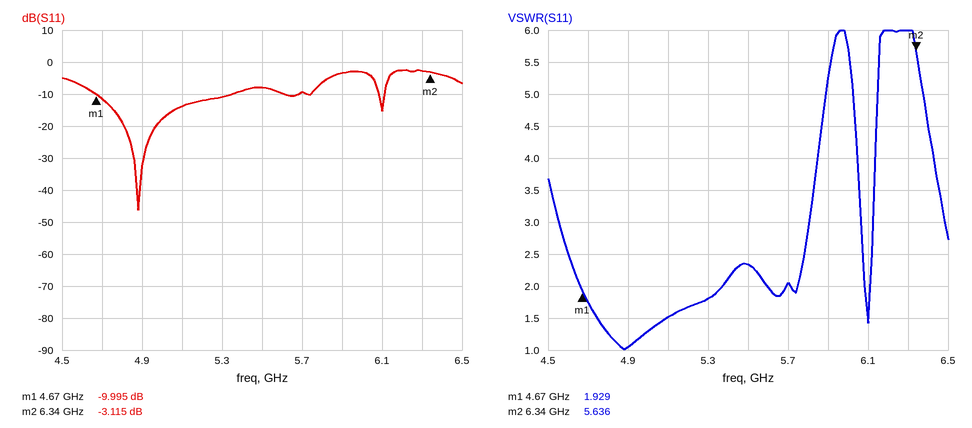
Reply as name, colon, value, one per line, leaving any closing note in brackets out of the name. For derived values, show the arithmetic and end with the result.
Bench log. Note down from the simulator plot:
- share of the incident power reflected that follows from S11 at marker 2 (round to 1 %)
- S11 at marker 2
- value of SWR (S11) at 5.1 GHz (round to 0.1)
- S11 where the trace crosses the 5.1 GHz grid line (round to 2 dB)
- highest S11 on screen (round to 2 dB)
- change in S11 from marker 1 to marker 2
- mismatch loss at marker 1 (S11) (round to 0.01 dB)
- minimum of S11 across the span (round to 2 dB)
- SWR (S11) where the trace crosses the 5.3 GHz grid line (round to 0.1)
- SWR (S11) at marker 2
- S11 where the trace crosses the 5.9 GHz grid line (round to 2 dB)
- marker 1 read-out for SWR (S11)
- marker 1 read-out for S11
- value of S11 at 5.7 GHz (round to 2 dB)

share of the incident power reflected that follows from S11 at marker 2: 10^(-3.115/10) ≈ 49 %
S11 at marker 2: -3.115 dB
value of SWR (S11) at 5.1 GHz: 1.5
S11 where the trace crosses the 5.1 GHz grid line: -14 dB
highest S11 on screen: -2 dB
change in S11 from marker 1 to marker 2: -3.115 − (-9.995) = 6.880 dB
mismatch loss at marker 1 (S11): −10 log10(1 − 10^(-9.995/10)) ≈ 0.46 dB
minimum of S11 across the span: -46 dB
SWR (S11) where the trace crosses the 5.3 GHz grid line: 1.8
SWR (S11) at marker 2: 5.636
S11 where the trace crosses the 5.9 GHz grid line: -4 dB
marker 1 read-out for SWR: 1.929
marker 1 read-out for S11: -9.995 dB
value of S11 at 5.7 GHz: -10 dB
